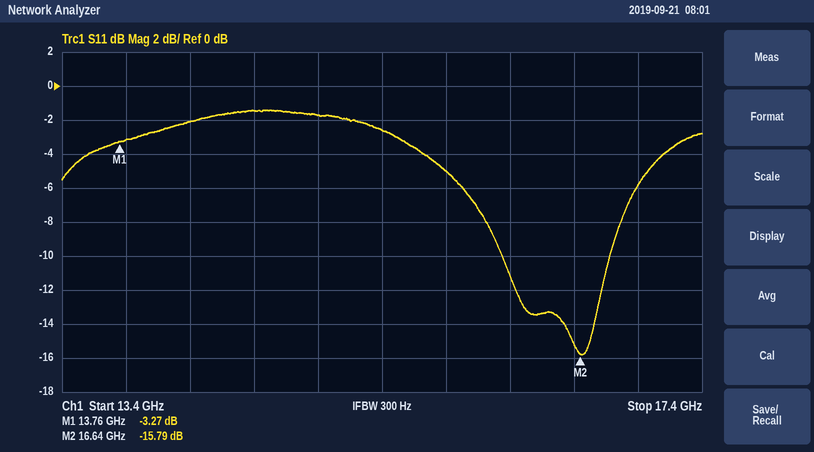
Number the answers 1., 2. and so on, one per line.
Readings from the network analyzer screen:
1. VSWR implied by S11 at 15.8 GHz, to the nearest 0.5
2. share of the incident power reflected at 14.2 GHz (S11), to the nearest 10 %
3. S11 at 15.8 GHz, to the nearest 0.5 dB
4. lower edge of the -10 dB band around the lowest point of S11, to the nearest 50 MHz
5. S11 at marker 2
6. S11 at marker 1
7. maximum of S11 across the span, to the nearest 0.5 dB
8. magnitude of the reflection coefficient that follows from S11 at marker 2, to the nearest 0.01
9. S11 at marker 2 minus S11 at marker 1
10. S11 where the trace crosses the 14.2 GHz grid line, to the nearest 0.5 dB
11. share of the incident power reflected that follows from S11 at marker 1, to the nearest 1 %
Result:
1. 3.5
2. 60 %
3. -5.0 dB
4. 16.15 GHz
5. -15.79 dB
6. -3.27 dB
7. -1.5 dB
8. 0.16
9. -12.52 dB
10. -2.0 dB
11. 47 %
